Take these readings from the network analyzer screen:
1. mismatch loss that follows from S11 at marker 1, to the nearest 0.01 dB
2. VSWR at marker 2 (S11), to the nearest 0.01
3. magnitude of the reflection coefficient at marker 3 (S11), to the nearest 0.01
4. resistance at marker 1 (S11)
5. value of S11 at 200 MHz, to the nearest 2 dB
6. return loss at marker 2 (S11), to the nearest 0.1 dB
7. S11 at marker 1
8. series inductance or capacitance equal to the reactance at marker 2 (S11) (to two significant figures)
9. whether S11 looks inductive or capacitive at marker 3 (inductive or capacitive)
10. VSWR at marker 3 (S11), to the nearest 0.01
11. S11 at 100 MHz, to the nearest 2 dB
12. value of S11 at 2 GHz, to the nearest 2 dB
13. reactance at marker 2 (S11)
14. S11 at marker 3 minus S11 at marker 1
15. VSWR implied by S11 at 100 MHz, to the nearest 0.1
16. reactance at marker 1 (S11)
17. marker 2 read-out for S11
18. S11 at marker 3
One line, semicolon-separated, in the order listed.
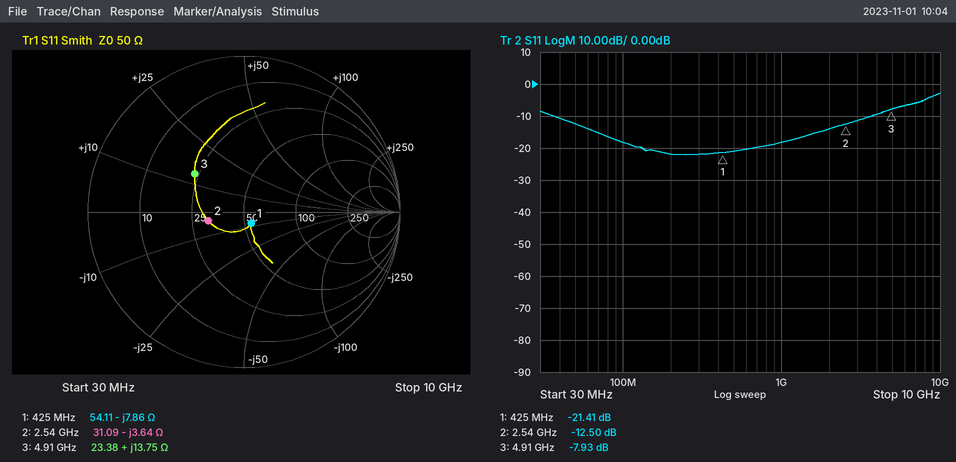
0.03 dB; 1.62; 0.40; 54.11 Ω; -22 dB; 12.5 dB; -21.41 dB; 17 pF; inductive; 2.34; -18 dB; -14 dB; -3.64 Ω; 13.48 dB; 1.3; -7.86 Ω; -12.50 dB; -7.93 dB
